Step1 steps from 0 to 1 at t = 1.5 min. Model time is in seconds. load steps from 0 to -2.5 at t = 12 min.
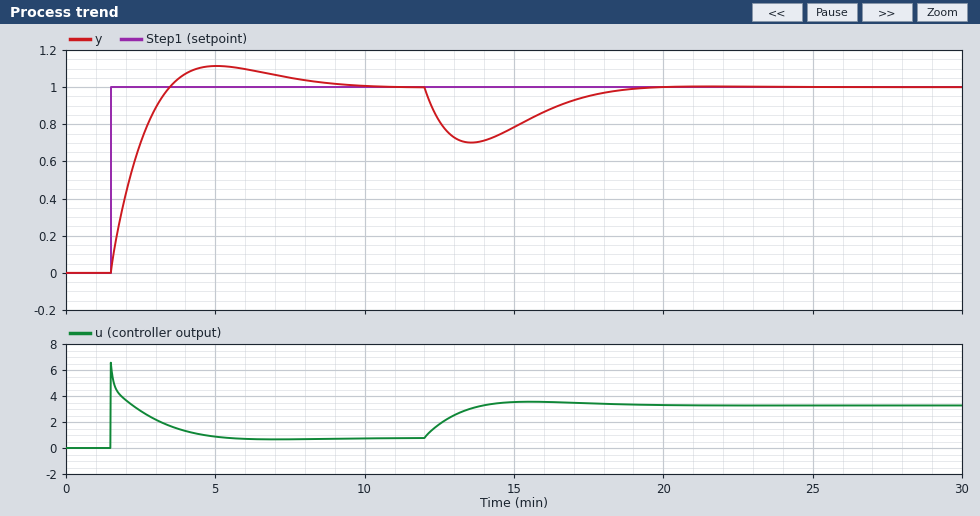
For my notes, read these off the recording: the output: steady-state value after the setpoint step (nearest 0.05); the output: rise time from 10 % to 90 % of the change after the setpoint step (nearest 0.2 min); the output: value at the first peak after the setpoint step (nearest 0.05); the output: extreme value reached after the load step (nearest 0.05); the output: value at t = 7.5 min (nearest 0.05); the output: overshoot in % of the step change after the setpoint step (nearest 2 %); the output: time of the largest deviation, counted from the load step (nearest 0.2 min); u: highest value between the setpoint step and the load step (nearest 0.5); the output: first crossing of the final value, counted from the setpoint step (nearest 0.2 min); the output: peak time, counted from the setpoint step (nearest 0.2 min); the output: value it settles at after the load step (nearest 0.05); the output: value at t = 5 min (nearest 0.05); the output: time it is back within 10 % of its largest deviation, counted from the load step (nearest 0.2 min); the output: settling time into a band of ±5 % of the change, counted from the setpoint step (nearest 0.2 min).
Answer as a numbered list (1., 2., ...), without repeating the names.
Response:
1. 1.00
2. 1.4 min
3. 1.10
4. 0.70
5. 1.05
6. 12 %
7. 1.6 min
8. 6.5
9. 2.0 min
10. 3.6 min
11. 1.00
12. 1.10
13. 6.0 min
14. 6.0 min
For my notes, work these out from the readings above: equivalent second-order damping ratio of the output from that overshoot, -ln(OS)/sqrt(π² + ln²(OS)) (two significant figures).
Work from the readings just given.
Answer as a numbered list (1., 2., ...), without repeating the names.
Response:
1. 0.56
